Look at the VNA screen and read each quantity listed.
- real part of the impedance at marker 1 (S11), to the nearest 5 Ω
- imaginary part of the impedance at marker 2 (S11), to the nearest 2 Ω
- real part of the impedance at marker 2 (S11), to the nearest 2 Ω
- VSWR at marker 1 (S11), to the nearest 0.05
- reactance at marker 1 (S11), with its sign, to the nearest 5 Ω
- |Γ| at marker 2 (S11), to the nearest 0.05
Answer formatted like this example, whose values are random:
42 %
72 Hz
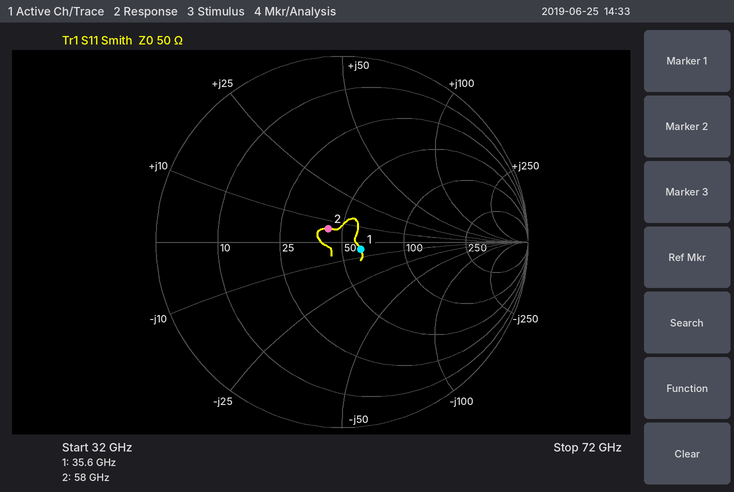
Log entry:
60 Ω
+6 Ω
42 Ω
1.25
-5 Ω
0.10
